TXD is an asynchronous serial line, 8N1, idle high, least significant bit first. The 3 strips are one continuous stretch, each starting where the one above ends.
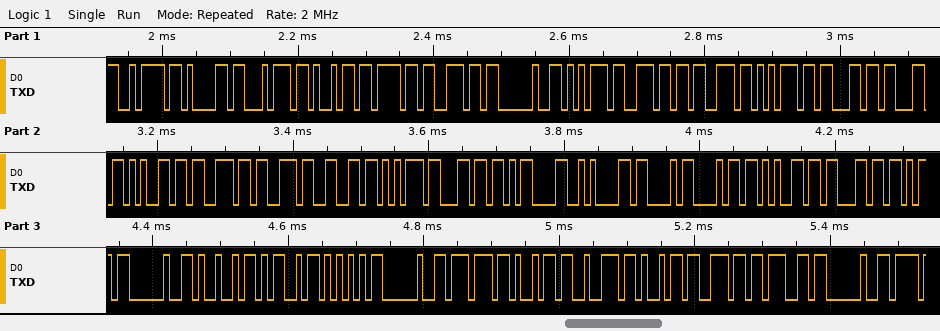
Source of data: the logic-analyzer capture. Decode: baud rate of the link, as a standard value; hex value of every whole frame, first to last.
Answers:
115200 baud
7A 61 74 69 6F 6E 20 75 6E 73 75 63 63 65 73 73 66 75 6C 0D 0A 43 68 65 63 6B 20 49 4D 55 20 77 69 72 69 6E 67 20
